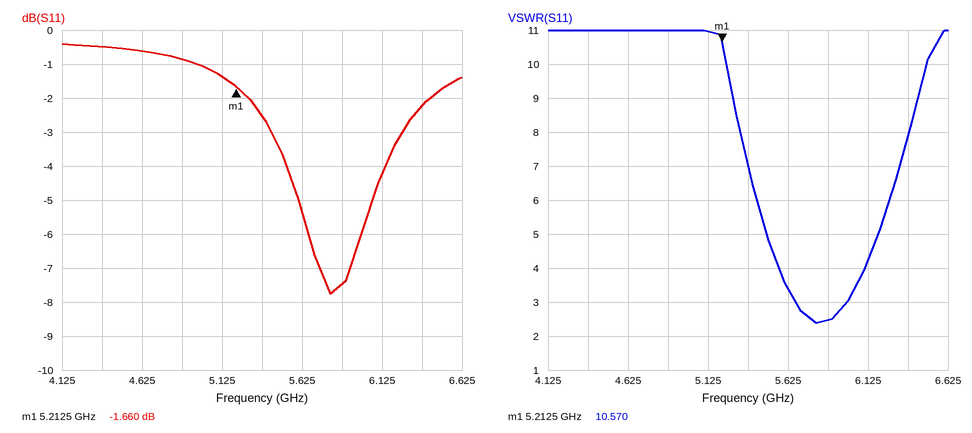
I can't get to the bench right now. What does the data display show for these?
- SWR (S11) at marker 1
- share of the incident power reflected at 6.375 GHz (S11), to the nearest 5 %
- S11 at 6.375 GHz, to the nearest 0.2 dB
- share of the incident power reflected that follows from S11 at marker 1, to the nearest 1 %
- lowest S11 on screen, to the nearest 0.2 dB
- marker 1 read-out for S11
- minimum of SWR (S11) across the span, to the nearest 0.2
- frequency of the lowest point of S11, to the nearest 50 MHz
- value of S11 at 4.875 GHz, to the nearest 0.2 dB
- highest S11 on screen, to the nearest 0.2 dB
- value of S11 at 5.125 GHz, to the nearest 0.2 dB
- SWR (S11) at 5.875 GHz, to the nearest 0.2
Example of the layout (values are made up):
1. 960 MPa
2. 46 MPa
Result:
1. 10.570
2. 60 %
3. -2.2 dB
4. 68 %
5. -7.8 dB
6. -1.660 dB
7. 2.4
8. 5.80 GHz
9. -0.8 dB
10. -0.4 dB
11. -1.4 dB
12. 2.4
